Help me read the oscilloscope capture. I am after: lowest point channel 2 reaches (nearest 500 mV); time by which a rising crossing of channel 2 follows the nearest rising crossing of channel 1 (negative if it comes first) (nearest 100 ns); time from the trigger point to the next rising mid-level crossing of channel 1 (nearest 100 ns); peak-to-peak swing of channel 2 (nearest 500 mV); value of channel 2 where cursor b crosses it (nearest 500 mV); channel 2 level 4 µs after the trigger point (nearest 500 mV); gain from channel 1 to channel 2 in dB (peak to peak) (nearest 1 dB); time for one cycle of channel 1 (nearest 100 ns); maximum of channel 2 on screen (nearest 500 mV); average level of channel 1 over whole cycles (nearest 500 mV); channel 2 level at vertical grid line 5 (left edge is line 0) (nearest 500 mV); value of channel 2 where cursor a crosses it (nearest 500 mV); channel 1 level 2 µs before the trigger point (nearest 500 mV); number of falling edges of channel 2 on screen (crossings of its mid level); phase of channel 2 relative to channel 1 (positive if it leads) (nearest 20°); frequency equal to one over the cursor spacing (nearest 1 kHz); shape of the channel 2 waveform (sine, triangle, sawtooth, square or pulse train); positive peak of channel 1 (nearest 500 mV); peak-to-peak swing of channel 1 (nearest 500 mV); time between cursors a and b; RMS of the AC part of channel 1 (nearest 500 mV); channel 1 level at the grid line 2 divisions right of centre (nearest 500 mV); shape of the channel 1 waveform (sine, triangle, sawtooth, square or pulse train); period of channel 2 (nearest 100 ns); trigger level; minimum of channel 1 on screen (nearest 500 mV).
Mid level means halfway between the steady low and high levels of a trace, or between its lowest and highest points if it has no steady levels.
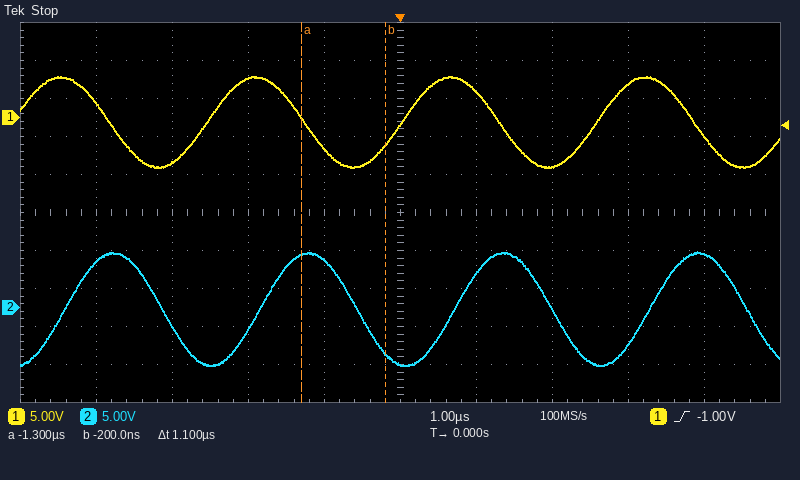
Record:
-7.5 V
+700 ns
2.6 µs
15.0 V
-6.0 V
7.0 V
2 dB
2.6 µs
7.5 V
-500 mV
-7.5 V
7.0 V
5.0 V
4
-100°
909 kHz
sine
5.5 V
12.0 V
1.1 µs
4.0 V
-6.5 V
sine
2.6 µs
-1.00 V
-6.5 V
